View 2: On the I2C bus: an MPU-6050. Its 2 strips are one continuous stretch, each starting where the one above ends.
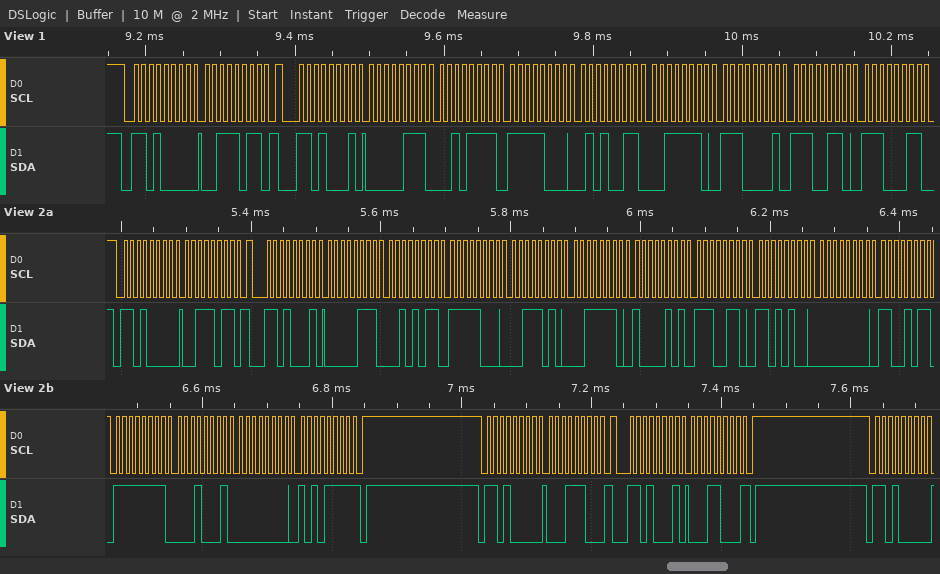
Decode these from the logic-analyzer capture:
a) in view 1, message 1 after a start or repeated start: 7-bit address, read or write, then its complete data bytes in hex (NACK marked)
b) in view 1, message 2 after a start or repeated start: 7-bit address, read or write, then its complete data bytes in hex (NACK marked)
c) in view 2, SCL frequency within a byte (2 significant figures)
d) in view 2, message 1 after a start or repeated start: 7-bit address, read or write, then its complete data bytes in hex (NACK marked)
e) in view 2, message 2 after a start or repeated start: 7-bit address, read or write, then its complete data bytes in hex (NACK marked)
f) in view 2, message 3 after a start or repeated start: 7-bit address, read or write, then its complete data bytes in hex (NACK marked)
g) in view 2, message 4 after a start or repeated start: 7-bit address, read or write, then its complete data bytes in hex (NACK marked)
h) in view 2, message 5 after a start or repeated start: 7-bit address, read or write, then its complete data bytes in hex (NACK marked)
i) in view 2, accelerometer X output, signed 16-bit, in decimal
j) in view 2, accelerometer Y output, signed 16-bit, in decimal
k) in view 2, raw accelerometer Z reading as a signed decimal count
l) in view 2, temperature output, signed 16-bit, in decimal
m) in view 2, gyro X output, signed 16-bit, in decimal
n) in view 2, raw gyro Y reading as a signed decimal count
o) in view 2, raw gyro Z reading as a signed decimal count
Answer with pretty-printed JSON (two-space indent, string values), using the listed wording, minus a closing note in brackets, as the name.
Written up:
{
  "in view 1, message 1 after a start or repeated start: 7-bit address, read or write, then its complete data bytes in hex": "0x68 write: 3B",
  "in view 1, message 2 after a start or repeated start: 7-bit address, read or write, then its complete data bytes in hex": "0x68 read: 07 2F F8 53 3E E1 E6 E3",
  "in view 2, SCL frequency within a byte": "100 kHz",
  "in view 2, message 1 after a start or repeated start: 7-bit address, read or write, then its complete data bytes in hex": "0x68 write: 3B",
  "in view 2, message 2 after a start or repeated start: 7-bit address, read or write, then its complete data bytes in hex": "0x68 read: 07 2B F8 3A 3E 85 E6 D4 00 CB FF 11 00 AF NACK",
  "in view 2, message 3 after a start or repeated start: 7-bit address, read or write, then its complete data bytes in hex": "0x68 write: 1C",
  "in view 2, message 4 after a start or repeated start: 7-bit address, read or write, then its complete data bytes in hex": "0x68 read: 18 NACK",
  "in view 2, message 5 after a start or repeated start: 7-bit address, read or write, then its complete data bytes in hex": "0x68 write",
  "in view 2, accelerometer X output, signed 16-bit, in decimal": "1835",
  "in view 2, accelerometer Y output, signed 16-bit, in decimal": "-1990",
  "in view 2, raw accelerometer Z reading as a signed decimal count": "16005",
  "in view 2, temperature output, signed 16-bit, in decimal": "-6444",
  "in view 2, gyro X output, signed 16-bit, in decimal": "203",
  "in view 2, raw gyro Y reading as a signed decimal count": "-239",
  "in view 2, raw gyro Z reading as a signed decimal count": "175"
}
